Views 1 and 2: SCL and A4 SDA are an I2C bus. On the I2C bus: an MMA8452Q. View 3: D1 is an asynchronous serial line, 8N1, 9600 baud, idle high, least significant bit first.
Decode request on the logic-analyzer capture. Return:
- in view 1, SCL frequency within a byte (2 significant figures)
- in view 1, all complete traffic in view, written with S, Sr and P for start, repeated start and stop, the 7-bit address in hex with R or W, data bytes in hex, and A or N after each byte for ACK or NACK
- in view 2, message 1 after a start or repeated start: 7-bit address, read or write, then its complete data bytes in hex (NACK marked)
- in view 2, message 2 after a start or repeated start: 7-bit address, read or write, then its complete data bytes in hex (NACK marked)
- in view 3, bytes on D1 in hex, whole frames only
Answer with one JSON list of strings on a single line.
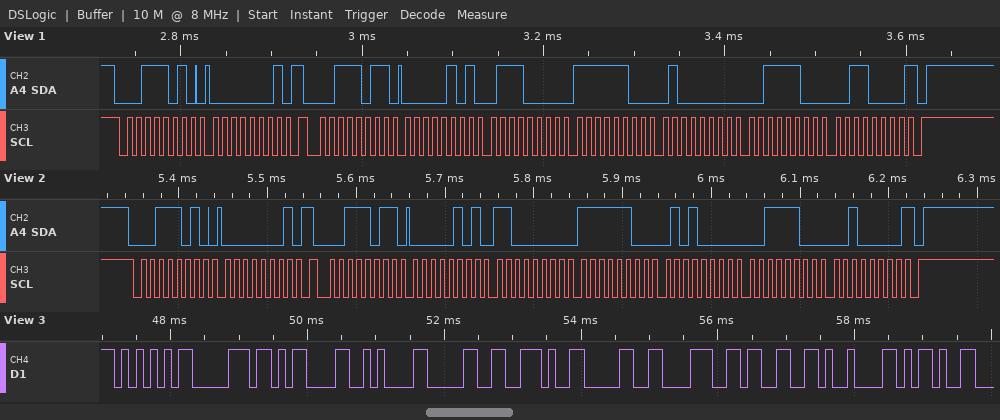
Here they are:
["100 kHz", "S 1DW A 01 A Sr 1DR A 05 A 70 A FC A 40 A 3C A 30 N P", "0x1D write: 01", "0x1D read: 05 C0 FC 50 3C 20 NACK", "55 70 0D 0A 30 2E 30 38 33 09 2D"]
